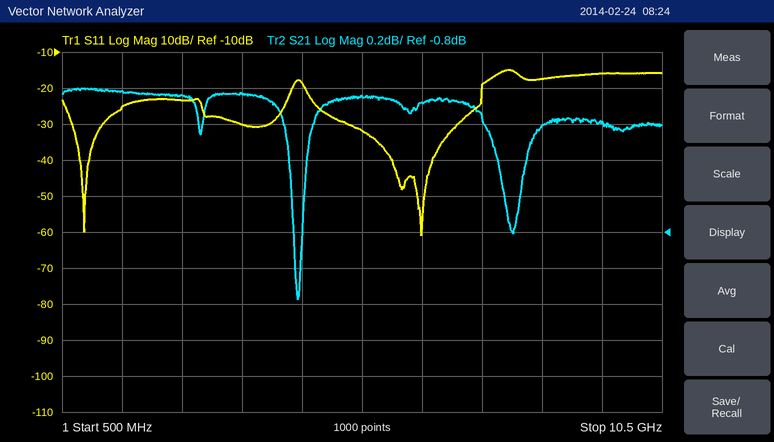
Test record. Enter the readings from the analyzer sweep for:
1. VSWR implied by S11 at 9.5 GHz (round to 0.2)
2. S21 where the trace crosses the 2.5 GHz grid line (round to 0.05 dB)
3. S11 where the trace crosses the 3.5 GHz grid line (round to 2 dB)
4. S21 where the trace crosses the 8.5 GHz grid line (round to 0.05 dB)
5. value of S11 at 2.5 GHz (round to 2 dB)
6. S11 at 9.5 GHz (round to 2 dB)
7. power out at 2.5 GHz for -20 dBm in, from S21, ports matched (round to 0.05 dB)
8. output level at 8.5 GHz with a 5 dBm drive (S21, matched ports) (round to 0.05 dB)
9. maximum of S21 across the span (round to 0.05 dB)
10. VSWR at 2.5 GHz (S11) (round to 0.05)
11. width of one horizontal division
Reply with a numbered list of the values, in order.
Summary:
1. 1.4
2. -0.05 dB
3. -30 dB
4. -0.20 dB
5. -24 dB
6. -16 dB
7. -20.05 dBm
8. 4.80 dBm
9. 0.00 dB
10. 1.15
11. 1 GHz
